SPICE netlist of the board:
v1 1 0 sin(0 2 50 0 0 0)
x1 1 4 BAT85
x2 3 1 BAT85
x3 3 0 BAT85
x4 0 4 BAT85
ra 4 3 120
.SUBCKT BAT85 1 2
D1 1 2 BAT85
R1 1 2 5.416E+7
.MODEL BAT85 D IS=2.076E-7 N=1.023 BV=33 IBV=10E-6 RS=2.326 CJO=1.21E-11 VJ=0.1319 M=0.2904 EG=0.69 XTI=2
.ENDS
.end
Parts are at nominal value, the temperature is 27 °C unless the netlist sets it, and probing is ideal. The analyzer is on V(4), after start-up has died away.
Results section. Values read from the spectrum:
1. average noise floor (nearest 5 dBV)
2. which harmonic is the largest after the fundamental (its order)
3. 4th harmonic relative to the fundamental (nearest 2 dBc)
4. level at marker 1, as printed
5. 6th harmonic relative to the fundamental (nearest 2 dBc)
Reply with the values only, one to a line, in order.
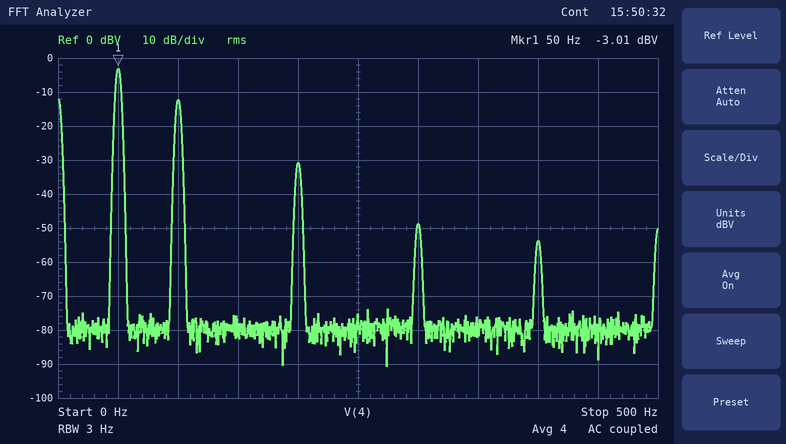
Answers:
-80 dBV
2
-28 dBc
-3.01 dBV
-46 dBc
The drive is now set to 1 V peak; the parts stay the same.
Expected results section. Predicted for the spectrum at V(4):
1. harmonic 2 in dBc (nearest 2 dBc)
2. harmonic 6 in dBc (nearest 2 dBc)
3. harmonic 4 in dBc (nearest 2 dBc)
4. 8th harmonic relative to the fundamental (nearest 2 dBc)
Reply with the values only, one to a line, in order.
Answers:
-12 dBc
-36 dBc
-44 dBc
-42 dBc
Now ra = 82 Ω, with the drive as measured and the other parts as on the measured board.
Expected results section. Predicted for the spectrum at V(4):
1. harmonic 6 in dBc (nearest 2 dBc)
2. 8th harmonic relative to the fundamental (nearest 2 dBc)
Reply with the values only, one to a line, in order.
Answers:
-48 dBc
-48 dBc
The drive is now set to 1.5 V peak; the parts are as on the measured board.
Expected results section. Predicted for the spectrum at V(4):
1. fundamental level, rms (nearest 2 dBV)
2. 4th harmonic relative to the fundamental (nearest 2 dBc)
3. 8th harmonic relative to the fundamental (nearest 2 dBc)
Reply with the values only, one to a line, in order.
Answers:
-6 dBV
-32 dBc
-42 dBc
